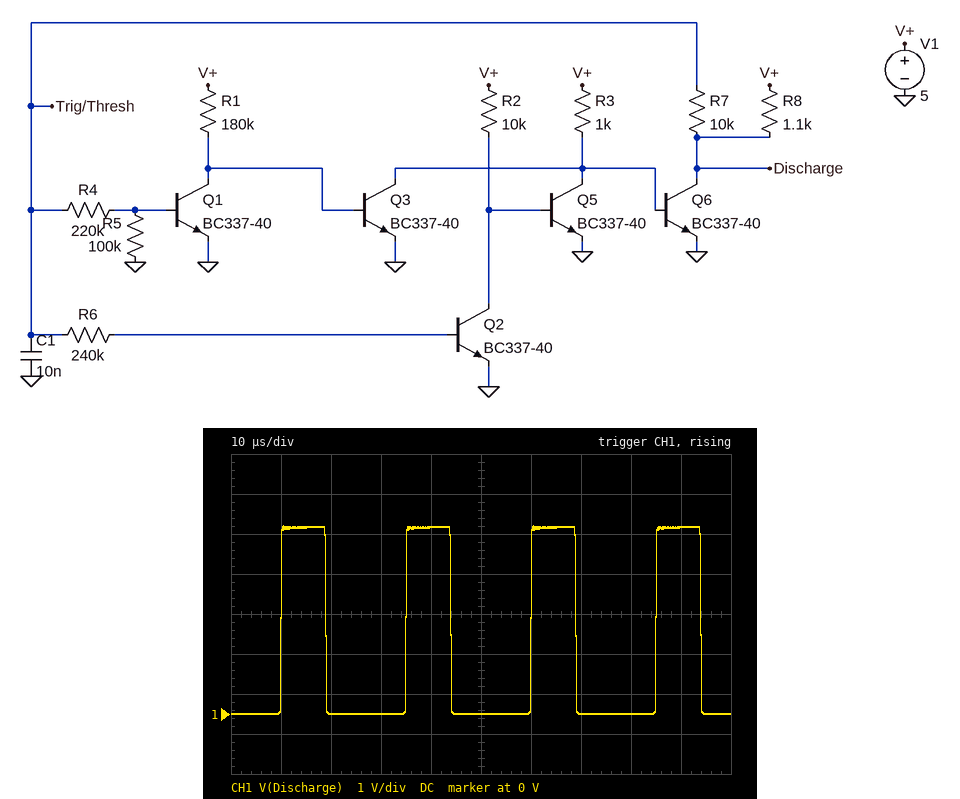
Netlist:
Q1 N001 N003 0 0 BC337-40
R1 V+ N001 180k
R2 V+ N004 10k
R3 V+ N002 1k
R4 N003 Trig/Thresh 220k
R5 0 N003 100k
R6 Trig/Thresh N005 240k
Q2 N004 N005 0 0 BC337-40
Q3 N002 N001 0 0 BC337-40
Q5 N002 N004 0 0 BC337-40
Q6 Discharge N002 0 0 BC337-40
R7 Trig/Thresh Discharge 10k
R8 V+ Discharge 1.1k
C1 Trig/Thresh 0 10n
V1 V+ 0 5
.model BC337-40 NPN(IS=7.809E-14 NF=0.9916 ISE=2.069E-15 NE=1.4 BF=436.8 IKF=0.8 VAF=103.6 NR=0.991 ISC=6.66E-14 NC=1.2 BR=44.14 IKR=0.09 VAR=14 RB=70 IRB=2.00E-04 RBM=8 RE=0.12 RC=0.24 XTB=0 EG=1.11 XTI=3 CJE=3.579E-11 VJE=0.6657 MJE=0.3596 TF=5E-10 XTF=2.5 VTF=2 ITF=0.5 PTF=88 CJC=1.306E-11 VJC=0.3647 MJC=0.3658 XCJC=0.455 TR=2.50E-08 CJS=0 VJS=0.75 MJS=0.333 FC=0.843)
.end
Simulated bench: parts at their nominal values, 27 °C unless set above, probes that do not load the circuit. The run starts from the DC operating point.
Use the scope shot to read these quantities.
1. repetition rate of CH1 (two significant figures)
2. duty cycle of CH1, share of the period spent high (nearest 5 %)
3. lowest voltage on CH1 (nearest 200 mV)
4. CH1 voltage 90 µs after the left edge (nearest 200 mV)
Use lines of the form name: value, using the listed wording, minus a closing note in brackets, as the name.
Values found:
repetition rate of CH1: 40 kHz
duty cycle of CH1, share of the period spent high: 35 %
lowest voltage on CH1: 0 V
CH1 voltage 90 µs after the left edge: 4.6 V
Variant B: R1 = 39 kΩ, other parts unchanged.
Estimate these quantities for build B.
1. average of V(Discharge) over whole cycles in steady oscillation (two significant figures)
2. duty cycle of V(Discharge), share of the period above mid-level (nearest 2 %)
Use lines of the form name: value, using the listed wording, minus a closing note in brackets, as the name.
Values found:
average of V(Discharge) over whole cycles in steady oscillation: 1.9 V
duty cycle of V(Discharge), share of the period above mid-level: 40 %
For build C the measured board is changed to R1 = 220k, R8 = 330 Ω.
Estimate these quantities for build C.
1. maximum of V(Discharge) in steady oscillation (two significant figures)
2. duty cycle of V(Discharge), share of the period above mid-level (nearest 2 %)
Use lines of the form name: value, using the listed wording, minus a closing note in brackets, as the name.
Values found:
maximum of V(Discharge) in steady oscillation: 4.9 V
duty cycle of V(Discharge), share of the period above mid-level: 34 %
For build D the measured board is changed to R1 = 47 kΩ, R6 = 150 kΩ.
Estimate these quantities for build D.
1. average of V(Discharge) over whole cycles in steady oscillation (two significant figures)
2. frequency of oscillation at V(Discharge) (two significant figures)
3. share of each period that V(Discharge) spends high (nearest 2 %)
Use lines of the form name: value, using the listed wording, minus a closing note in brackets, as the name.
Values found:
average of V(Discharge) over whole cycles in steady oscillation: 1.9 V
frequency of oscillation at V(Discharge): 49 kHz
share of each period that V(Discharge) spends high: 40 %
